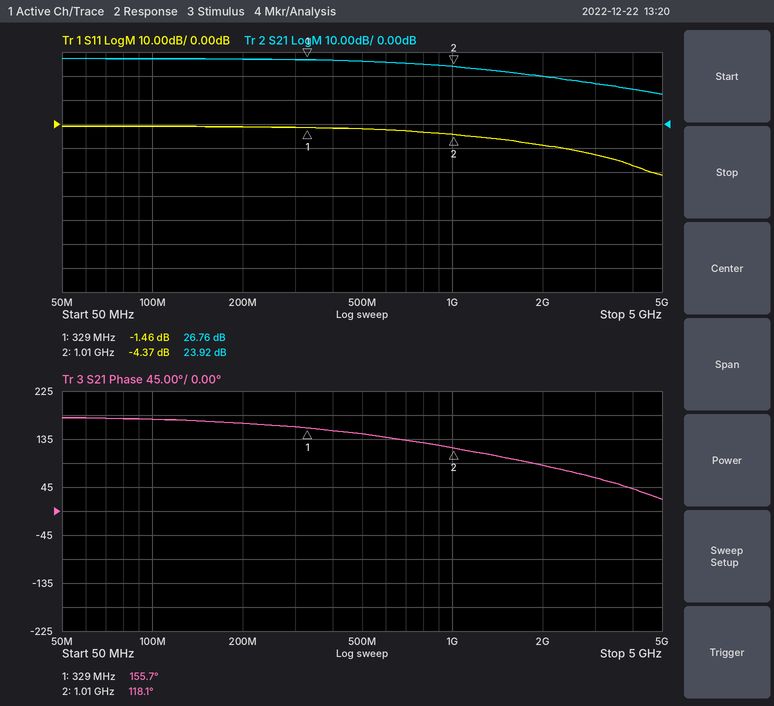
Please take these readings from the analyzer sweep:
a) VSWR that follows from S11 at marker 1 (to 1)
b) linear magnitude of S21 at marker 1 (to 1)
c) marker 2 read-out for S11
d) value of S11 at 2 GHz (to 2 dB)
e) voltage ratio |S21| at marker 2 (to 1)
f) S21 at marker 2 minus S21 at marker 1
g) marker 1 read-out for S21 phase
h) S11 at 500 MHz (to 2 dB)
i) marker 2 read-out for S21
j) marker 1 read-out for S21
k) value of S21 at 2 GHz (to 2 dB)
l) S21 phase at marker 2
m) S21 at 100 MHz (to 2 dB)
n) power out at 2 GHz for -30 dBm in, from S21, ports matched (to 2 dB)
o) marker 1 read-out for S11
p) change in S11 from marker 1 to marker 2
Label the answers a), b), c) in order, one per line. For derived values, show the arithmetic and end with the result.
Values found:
a) (1 + 0.8453)/(1 − 0.8453) ≈ 12
b) 10^(26.76/20) ≈ 22
c) -4.37 dB
d) -8 dB
e) 10^(23.92/20) ≈ 16
f) 23.92 − (26.76) = -2.84 dB
g) 155.7°
h) -2 dB
i) 23.92 dB
j) 26.76 dB
k) 20 dB
l) 118.1°
m) 28 dB
n) -30 dBm + (20 dB) = -10 dBm
o) -1.46 dB
p) -4.37 − (-1.46) = -2.91 dB
